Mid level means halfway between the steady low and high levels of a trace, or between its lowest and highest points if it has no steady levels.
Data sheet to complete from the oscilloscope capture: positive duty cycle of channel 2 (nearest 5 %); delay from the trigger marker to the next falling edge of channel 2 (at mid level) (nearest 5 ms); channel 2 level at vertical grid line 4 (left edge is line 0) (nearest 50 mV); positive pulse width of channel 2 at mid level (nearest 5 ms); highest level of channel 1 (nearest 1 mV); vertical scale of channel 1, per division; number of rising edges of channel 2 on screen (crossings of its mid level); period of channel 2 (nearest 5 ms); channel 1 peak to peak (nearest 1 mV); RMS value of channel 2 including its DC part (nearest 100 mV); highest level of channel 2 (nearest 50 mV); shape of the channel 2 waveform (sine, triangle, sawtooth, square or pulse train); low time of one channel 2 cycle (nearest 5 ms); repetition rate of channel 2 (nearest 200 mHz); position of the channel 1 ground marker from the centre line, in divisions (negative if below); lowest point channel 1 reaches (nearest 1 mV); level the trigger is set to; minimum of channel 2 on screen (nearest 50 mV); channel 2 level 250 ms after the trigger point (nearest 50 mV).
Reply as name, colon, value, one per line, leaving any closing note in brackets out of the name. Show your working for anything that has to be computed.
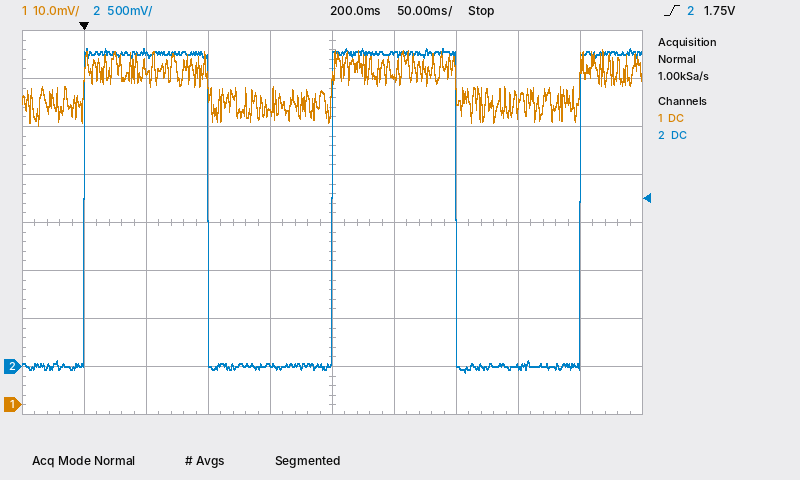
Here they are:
positive duty cycle of channel 2: 100 ms / 200 ms ≈ 50 %
delay from the trigger marker to the next falling edge of channel 2 (at mid level): 100 ms
channel 2 level at vertical grid line 4 (left edge is line 0): 0 mV
positive pulse width of channel 2 at mid level: 100 ms
highest level of channel 1: 74 mV
vertical scale of channel 1, per division: 10 mV
number of rising edges of channel 2 on screen: 3
period of channel 2: 200 ms
channel 1 peak to peak: 74 mV − (58 mV) = 16 mV
RMS value of channel 2 including its DC part: √(0.5 × (3.30 V)² + 0.5 × (-50 mV)²) ≈ 2.3 V
highest level of channel 2: 3.30 V
shape of the channel 2 waveform: square
low time of one channel 2 cycle: 100 ms
repetition rate of channel 2: 1 / 200 ms ≈ 5.0 Hz
position of the channel 1 ground marker from the centre line, in divisions: -3.8 div
lowest point channel 1 reaches: 58 mV
level the trigger is set to: 1.75 V
minimum of channel 2 on screen: -50 mV
channel 2 level 250 ms after the trigger point: 3.25 V
